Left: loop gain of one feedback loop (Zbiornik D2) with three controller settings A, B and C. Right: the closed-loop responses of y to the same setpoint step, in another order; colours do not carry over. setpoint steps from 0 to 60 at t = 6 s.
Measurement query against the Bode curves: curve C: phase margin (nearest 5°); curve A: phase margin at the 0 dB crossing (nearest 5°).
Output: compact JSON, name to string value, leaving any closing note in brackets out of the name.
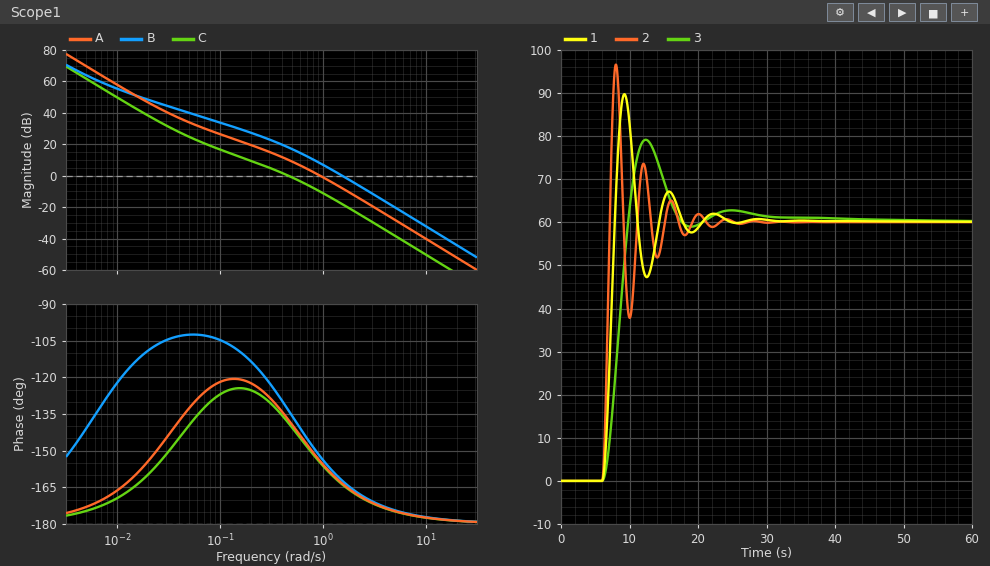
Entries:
{"curve C: phase margin": "40°", "curve A: phase margin at the 0 dB crossing": "25°"}
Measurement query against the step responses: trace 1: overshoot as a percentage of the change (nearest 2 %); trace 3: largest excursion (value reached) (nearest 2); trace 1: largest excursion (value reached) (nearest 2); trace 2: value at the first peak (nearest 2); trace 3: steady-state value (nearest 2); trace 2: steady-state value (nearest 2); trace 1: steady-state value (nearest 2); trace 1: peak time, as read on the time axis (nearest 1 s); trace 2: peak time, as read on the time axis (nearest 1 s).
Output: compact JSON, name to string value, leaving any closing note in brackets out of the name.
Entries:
{"trace 1: overshoot as a percentage of the change": "50 %", "trace 3: largest excursion (value reached)": "80", "trace 1: largest excursion (value reached)": "90", "trace 2: value at the first peak": "96", "trace 3: steady-state value": "60", "trace 2: steady-state value": "60", "trace 1: steady-state value": "60", "trace 1: peak time, as read on the time axis": "9 s", "trace 2: peak time, as read on the time axis": "8 s"}
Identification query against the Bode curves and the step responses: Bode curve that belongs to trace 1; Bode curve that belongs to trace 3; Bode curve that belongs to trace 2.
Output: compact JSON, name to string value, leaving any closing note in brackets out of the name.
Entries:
{"Bode curve that belongs to trace 1": "A", "Bode curve that belongs to trace 3": "C", "Bode curve that belongs to trace 2": "B"}
